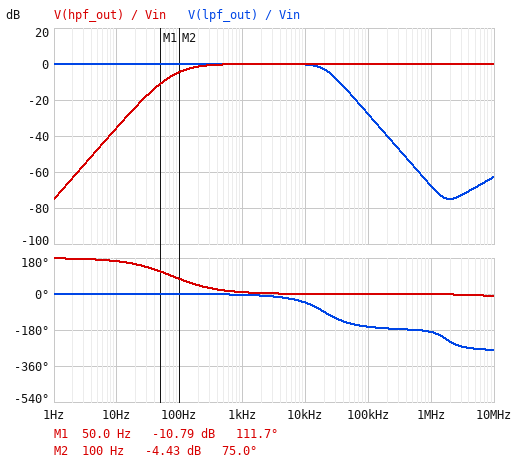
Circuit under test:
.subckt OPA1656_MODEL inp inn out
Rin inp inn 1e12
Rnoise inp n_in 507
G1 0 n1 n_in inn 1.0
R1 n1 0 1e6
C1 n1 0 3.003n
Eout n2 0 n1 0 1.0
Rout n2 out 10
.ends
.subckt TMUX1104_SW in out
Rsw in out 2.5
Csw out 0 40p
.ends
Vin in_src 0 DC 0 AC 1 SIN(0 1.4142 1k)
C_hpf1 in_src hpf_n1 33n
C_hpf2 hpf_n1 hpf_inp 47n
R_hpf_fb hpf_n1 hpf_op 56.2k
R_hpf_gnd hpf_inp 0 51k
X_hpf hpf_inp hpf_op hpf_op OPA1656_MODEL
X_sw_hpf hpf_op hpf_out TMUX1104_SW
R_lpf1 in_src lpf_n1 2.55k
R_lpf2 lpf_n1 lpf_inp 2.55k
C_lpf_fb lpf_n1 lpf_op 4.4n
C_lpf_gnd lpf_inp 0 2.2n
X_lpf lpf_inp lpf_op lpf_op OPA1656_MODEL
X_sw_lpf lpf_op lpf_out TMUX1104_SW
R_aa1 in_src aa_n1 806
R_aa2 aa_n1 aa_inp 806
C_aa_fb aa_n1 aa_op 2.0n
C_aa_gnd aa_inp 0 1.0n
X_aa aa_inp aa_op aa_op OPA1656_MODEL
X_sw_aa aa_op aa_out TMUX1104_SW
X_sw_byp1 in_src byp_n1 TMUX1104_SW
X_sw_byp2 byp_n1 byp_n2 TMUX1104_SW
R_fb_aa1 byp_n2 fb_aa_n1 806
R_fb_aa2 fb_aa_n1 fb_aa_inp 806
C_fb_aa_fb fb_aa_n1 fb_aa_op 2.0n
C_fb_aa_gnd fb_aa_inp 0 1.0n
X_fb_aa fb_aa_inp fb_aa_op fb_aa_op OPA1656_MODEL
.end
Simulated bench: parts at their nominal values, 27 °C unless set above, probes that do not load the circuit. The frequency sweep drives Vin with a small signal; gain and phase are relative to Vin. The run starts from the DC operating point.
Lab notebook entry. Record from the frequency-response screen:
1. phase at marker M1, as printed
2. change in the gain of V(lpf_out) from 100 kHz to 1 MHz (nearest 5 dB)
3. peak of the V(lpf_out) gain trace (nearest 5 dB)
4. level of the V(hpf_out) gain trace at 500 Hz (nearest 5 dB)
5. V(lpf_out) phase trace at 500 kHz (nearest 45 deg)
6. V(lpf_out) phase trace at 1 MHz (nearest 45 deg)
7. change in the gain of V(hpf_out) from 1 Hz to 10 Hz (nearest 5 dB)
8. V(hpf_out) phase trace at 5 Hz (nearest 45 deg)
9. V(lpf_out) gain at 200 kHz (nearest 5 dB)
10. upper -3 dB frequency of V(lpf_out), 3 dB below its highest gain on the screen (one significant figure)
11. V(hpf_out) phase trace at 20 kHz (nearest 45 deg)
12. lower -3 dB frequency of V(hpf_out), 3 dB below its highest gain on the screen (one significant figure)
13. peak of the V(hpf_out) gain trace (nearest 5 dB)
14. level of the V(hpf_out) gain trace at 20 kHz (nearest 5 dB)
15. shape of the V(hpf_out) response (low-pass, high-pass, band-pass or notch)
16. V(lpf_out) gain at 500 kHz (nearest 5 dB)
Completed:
111.7 deg
-40 dB
0 dB
0 dB
-180 deg
-180 deg
40 dB
180 deg
-40 dB
20 kHz
0 deg
100 Hz
0 dB
0 dB
high-pass
-55 dB
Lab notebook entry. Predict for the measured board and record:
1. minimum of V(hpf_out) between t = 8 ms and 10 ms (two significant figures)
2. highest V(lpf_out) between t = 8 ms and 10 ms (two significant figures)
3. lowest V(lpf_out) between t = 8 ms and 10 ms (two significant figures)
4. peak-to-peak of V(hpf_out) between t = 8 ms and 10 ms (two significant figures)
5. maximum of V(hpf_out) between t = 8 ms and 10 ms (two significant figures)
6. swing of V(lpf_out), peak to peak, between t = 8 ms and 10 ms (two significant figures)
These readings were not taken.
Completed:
-1.4 V
1.4 V
-1.4 V
2.8 V
1.4 V
2.8 V
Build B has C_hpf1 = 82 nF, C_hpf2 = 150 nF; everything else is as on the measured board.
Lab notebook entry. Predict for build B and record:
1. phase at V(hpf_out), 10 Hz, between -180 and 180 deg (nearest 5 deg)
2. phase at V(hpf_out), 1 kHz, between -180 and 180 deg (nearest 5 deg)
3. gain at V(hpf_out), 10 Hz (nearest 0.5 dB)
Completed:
135 deg
5 deg
-18.5 dB
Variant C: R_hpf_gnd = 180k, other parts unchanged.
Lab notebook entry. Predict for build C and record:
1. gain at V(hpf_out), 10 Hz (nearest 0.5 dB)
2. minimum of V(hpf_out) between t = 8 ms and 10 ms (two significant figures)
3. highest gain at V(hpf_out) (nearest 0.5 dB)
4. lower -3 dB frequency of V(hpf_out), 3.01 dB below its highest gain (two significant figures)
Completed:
-24.0 dB
-1.4 V
0.5 dB
35 Hz
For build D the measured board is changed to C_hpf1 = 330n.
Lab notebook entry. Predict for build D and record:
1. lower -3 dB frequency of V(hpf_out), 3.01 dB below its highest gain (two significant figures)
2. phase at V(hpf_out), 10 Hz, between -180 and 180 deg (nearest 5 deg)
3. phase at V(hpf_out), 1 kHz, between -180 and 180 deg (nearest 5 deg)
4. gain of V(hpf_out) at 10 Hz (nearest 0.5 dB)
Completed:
68 Hz
120 deg
5 deg
-19.0 dB
